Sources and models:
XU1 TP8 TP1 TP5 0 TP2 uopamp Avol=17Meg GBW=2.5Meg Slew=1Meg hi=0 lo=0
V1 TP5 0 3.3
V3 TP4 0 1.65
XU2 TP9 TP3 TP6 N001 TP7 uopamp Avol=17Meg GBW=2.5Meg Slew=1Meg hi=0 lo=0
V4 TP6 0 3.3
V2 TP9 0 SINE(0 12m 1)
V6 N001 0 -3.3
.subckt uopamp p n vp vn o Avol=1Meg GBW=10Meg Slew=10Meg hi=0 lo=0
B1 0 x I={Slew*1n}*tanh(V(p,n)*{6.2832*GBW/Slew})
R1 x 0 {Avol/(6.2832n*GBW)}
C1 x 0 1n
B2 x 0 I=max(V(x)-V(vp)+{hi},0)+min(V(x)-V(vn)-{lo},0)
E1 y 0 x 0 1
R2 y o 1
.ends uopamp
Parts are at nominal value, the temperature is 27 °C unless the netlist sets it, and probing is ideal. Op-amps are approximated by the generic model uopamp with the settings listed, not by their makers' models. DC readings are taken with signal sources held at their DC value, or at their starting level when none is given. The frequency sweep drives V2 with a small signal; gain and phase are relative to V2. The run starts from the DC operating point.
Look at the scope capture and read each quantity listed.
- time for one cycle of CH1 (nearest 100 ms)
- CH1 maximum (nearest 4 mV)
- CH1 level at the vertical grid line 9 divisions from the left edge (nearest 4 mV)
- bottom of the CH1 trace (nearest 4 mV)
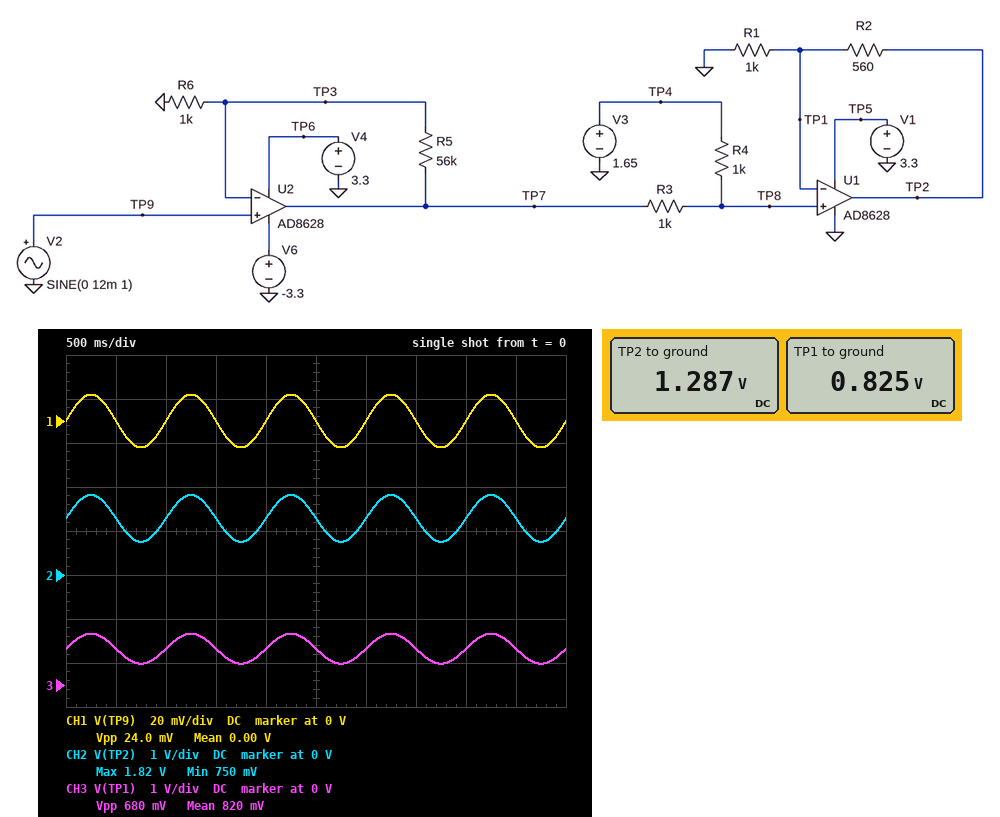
1.0 s
12 mV
0 V
-12 mV
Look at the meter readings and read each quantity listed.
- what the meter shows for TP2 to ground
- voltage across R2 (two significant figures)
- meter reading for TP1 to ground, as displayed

1.287 V
460 mV
0.825 V
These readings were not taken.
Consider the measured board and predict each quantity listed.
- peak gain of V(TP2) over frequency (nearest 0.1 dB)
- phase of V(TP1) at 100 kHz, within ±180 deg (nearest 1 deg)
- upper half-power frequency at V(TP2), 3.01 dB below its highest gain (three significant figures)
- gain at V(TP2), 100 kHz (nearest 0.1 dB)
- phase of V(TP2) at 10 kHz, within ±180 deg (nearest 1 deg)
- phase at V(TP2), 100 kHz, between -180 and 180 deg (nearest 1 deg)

33.0 dB
-70 deg
43.8 kHz
25.0 dB
-13 deg
-70 deg
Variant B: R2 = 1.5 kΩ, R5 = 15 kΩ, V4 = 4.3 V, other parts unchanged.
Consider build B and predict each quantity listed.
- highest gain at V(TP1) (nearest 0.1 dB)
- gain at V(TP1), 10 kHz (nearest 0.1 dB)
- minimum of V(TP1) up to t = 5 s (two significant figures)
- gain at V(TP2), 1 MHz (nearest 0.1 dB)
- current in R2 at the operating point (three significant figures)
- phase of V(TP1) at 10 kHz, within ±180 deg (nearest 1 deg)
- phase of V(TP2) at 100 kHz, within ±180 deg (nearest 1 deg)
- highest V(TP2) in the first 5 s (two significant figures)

18.1 dB
18.0 dB
730 mV
6.8 dB
825 µA
-4 deg
-38 deg
2.3 V
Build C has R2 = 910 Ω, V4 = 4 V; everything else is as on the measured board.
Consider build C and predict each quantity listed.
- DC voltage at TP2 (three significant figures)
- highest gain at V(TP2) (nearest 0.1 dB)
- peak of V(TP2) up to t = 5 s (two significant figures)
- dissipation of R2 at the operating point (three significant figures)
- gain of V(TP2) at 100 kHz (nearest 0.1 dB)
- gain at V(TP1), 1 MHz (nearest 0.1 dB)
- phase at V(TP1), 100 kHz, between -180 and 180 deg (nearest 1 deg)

1.58 V
34.7 dB
2.2 V
619 µW
26.8 dB
-0.1 dB
-71 deg
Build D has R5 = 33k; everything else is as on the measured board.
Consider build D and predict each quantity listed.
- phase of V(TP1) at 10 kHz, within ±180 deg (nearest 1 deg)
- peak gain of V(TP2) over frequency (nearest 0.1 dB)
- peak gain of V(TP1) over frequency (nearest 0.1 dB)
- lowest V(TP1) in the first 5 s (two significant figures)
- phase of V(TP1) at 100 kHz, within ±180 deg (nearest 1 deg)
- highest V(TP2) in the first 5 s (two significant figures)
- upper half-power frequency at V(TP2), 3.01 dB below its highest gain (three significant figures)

-8 deg
28.5 dB
24.6 dB
620 mV
-57 deg
1.6 V
73.3 kHz
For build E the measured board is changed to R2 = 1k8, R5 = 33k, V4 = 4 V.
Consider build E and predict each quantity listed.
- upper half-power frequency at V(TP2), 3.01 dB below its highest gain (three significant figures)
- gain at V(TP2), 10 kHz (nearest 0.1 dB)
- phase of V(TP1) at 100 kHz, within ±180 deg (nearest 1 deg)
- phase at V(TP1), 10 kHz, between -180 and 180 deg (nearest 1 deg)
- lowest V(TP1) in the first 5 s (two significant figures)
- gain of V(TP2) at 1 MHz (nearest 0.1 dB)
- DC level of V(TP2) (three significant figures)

73.0 kHz
33.5 dB
-60 deg
-8 deg
620 mV
7.3 dB
2.31 V
